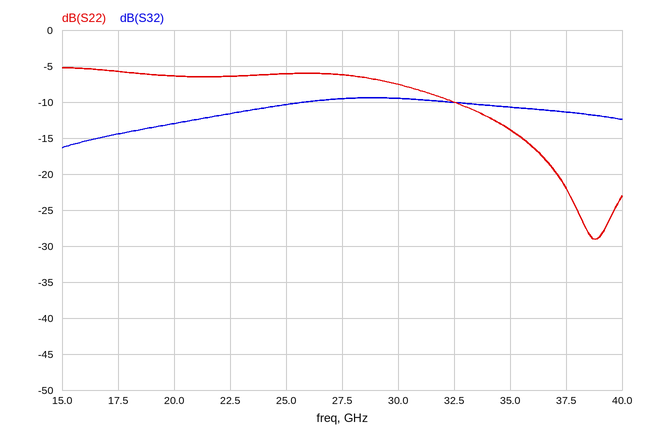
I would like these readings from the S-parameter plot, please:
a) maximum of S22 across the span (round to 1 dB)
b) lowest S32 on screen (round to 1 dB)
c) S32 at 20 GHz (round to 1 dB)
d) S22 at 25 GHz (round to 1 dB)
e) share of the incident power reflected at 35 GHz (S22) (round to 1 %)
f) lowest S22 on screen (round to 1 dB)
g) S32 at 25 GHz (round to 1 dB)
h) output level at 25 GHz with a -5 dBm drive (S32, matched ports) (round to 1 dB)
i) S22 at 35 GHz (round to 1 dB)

-5 dB
-16 dB
-13 dB
-6 dB
4 %
-29 dB
-10 dB
-15 dBm
-14 dB
